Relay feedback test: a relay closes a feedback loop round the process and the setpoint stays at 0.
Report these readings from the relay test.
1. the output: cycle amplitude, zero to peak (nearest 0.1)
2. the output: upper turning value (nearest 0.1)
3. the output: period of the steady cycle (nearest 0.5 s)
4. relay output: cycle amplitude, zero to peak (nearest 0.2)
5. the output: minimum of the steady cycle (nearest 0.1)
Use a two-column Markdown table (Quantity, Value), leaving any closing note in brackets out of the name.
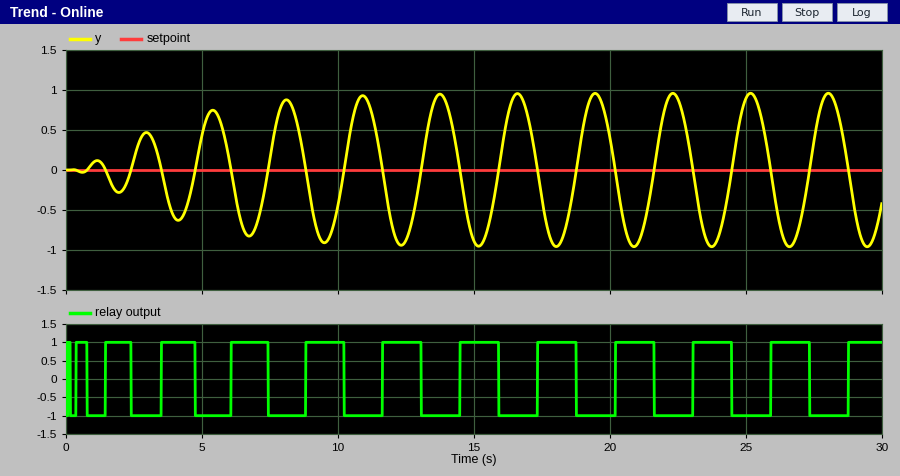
| Quantity | Value |
|---|---|
| the output: cycle amplitude, zero to peak | 1.0 |
| the output: upper turning value | 1.0 |
| the output: period of the steady cycle | 3.0 s |
| relay output: cycle amplitude, zero to peak | 1.0 |
| the output: minimum of the steady cycle | -1.0 |
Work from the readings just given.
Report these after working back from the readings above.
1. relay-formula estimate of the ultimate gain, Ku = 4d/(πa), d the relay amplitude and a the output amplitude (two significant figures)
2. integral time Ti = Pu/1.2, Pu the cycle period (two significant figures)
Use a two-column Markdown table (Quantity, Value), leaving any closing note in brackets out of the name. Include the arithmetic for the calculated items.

| Quantity | Value |
|---|---|
| relay-formula estimate of the ultimate gain, Ku = 4d/(πa), d the relay amplitude and a the output amplitude | 4 × 1 / (π × 1) = 1.3 |
| integral time Ti = Pu/1.2, Pu the cycle period | 3 / 1.2 = 2.5 s |
